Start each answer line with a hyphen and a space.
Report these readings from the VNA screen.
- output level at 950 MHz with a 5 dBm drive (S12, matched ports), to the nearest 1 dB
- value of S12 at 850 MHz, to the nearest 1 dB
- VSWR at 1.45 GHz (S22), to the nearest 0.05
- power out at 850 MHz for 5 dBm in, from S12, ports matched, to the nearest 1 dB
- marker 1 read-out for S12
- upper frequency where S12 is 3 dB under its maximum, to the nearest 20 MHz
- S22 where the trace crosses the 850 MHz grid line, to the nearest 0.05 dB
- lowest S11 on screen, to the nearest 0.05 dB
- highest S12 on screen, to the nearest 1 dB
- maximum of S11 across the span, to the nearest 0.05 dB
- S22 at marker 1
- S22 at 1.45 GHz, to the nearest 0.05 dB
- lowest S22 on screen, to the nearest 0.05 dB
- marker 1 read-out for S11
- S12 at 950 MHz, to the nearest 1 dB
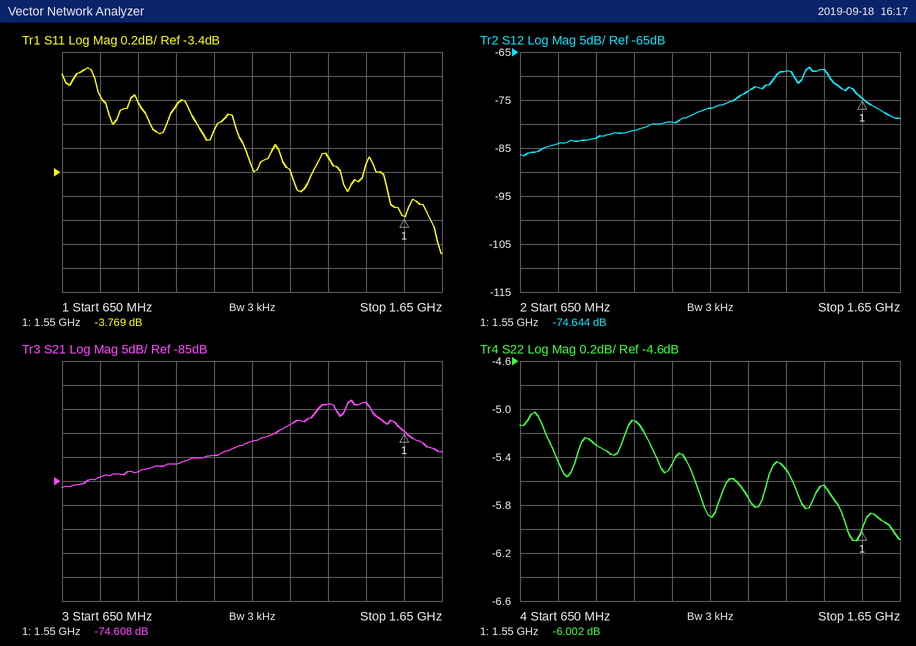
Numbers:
- -76 dBm
- -83 dB
- 3.20
- -78 dBm
- -74.644 dB
- 1.48 GHz
- -5.30 dB
- -4.10 dB
- -68 dB
- -2.55 dB
- -6.002 dB
- -5.65 dB
- -6.10 dB
- -3.769 dB
- -81 dB
